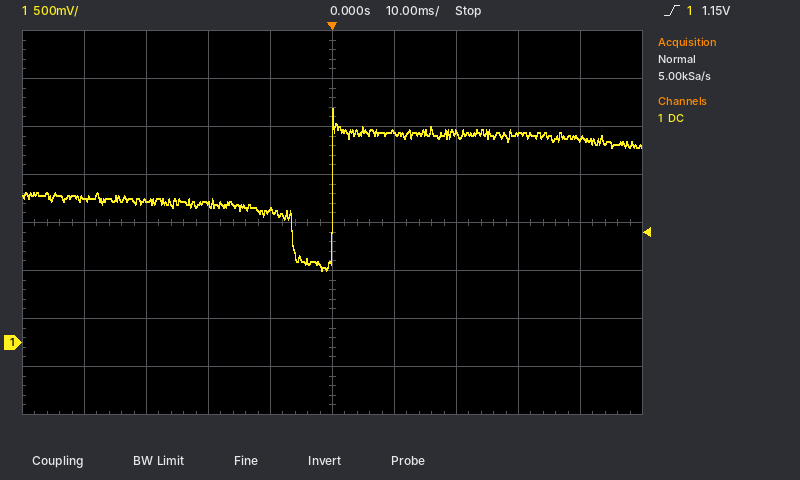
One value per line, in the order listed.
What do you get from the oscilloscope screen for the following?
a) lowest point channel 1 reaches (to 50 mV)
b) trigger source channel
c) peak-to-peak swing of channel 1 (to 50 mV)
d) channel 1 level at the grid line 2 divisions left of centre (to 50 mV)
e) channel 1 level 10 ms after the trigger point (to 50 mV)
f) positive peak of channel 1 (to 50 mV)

750 mV
channel 1
1.70 V
1.45 V
2.20 V
2.45 V
